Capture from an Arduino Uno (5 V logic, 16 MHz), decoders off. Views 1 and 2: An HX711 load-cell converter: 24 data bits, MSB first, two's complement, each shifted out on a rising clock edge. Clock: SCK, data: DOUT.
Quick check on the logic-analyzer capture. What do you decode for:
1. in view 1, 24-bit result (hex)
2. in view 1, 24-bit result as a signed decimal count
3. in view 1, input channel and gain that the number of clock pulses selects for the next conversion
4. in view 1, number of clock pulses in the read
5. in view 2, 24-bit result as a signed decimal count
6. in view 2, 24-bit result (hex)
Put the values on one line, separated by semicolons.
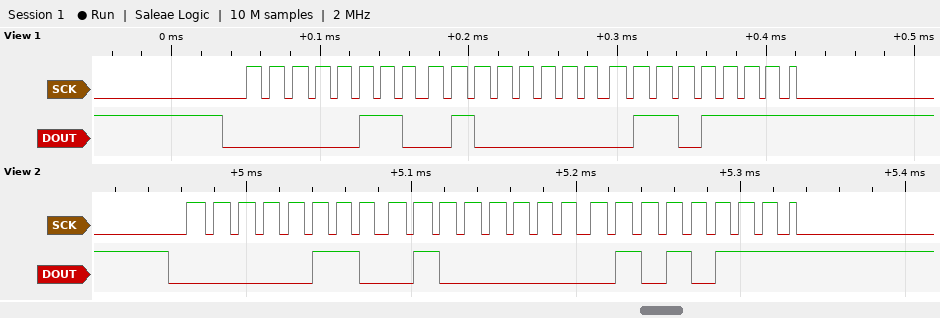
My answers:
0x06406F; 409711; channel A, gain 128; 25; 409687; 0x064057
